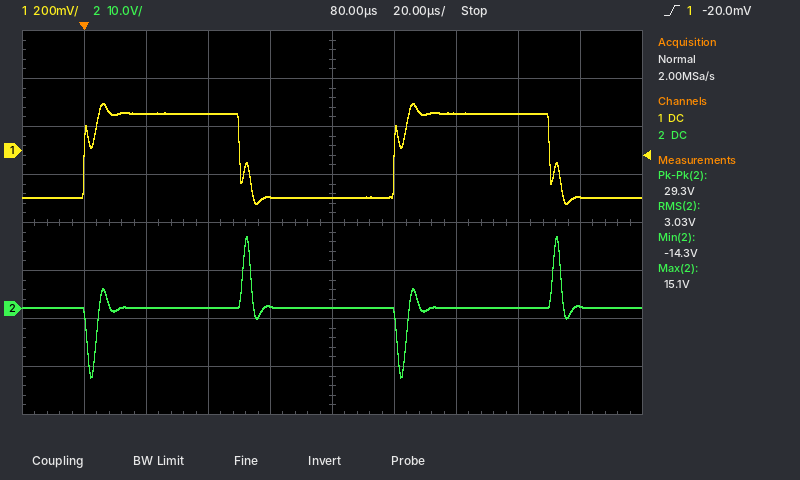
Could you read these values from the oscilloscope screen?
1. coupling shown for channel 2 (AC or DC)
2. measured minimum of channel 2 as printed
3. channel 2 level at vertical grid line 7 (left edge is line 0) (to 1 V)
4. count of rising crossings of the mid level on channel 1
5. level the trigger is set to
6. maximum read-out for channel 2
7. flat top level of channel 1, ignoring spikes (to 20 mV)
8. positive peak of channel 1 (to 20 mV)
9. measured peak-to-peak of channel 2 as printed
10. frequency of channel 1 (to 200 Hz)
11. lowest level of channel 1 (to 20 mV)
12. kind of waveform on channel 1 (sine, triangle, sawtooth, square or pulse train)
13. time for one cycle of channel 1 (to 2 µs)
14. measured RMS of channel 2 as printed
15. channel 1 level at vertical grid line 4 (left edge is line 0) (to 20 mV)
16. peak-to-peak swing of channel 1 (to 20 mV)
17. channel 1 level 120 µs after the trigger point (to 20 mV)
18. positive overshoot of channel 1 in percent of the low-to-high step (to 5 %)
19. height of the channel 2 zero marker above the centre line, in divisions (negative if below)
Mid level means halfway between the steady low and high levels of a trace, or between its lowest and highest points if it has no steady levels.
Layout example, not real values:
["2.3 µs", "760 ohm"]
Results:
["DC", "-14.3 V", "0 V", "2", "-20.0 mV", "15.1 V", "160 mV", "200 mV", "29.3 V", "10.0 kHz", "-220 mV", "square", "100 µs", "3.03 V", "-200 mV", "420 mV", "160 mV", "10 %", "-1.8 div"]
